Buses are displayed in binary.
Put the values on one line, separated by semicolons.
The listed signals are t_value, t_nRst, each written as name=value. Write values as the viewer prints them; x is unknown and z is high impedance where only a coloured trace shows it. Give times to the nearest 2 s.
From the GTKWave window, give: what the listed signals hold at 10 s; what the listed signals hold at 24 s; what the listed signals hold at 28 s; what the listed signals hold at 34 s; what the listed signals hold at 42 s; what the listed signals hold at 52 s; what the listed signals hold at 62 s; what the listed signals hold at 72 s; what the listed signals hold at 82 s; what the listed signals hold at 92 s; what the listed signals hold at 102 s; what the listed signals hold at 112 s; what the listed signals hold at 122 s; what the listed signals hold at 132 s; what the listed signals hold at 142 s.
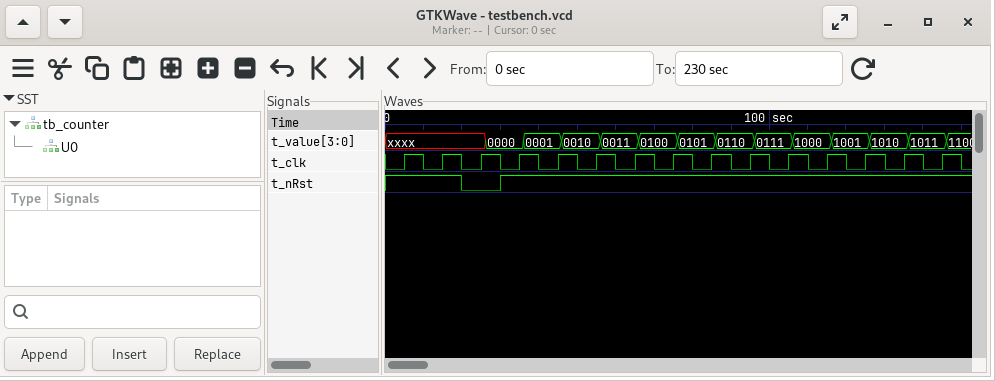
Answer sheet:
t_value=xxxx, t_nRst=1; t_value=xxxx, t_nRst=0; t_value=0000, t_nRst=0; t_value=0000, t_nRst=1; t_value=0001, t_nRst=1; t_value=0010, t_nRst=1; t_value=0011, t_nRst=1; t_value=0100, t_nRst=1; t_value=0101, t_nRst=1; t_value=0110, t_nRst=1; t_value=0111, t_nRst=1; t_value=1000, t_nRst=1; t_value=1001, t_nRst=1; t_value=1010, t_nRst=1; t_value=1011, t_nRst=1
